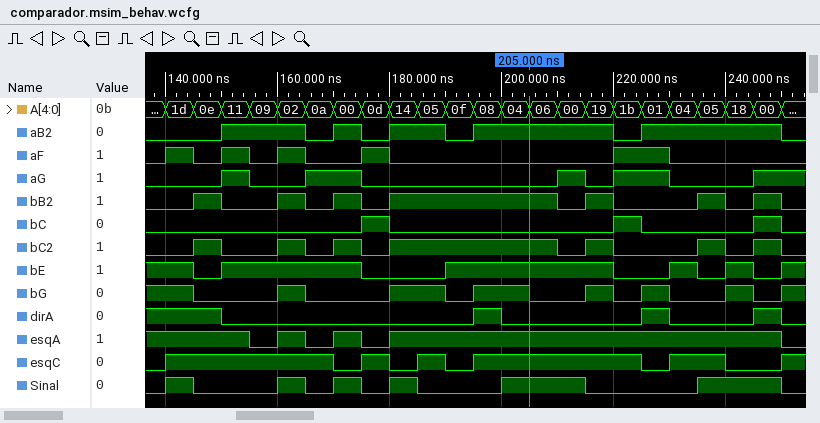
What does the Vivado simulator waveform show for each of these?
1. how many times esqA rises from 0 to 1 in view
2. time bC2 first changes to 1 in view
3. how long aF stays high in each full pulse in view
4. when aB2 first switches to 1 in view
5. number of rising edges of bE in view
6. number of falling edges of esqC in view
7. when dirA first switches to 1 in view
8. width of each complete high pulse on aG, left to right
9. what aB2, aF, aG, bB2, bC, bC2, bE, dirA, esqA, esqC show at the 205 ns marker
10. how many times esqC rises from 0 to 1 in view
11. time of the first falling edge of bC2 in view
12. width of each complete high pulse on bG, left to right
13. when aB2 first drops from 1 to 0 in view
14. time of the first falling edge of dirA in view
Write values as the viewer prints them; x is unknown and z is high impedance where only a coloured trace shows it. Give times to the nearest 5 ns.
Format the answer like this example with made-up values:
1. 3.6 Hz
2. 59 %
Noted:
1. 3
2. 145 ns
3. 5 ns, 5 ns, 5 ns, 5 ns, 10 ns
4. 150 ns
5. 5
6. 5
7. 195 ns
8. 5 ns, 10 ns, 5 ns, 10 ns
9. aB2=1, aF=0, aG=0, bB2=1, bC=0, bC2=1, bE=1, dirA=0, esqA=1, esqC=1
10. 6
11. 150 ns
12. 5 ns, 10 ns, 10 ns, 5 ns, 5 ns, 5 ns
13. 165 ns
14. 150 ns
